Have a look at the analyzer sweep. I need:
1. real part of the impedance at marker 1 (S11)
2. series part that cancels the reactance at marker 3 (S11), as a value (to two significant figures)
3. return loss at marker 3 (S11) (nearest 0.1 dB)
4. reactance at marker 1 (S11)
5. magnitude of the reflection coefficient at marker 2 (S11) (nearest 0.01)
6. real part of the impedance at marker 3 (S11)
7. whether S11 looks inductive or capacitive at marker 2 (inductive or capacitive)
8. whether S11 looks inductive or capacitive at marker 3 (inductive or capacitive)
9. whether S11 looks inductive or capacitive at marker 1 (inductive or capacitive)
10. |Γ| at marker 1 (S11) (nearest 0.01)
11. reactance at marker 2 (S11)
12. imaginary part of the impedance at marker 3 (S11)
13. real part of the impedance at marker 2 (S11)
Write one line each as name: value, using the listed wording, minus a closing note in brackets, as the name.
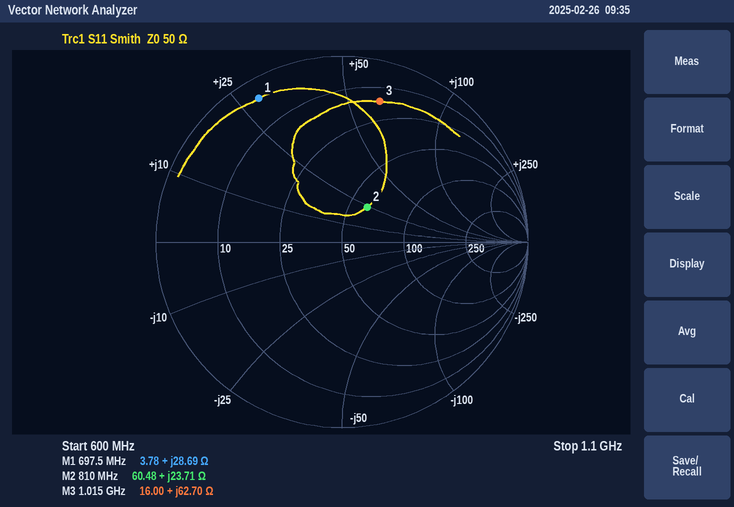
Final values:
real part of the impedance at marker 1: 3.78 Ω
series part that cancels the reactance at marker 3 (S11), as a value: 2.5 pF
return loss at marker 3 (S11): 2.1 dB
reactance at marker 1: +28.69 Ω
magnitude of the reflection coefficient at marker 2 (S11): 0.23
real part of the impedance at marker 3: 16.00 Ω
whether S11 looks inductive or capacitive at marker 2: inductive
whether S11 looks inductive or capacitive at marker 3: inductive
whether S11 looks inductive or capacitive at marker 1: inductive
|Γ| at marker 1 (S11): 0.89
reactance at marker 2: +23.71 Ω
imaginary part of the impedance at marker 3: +62.70 Ω
real part of the impedance at marker 2: 60.48 Ω
